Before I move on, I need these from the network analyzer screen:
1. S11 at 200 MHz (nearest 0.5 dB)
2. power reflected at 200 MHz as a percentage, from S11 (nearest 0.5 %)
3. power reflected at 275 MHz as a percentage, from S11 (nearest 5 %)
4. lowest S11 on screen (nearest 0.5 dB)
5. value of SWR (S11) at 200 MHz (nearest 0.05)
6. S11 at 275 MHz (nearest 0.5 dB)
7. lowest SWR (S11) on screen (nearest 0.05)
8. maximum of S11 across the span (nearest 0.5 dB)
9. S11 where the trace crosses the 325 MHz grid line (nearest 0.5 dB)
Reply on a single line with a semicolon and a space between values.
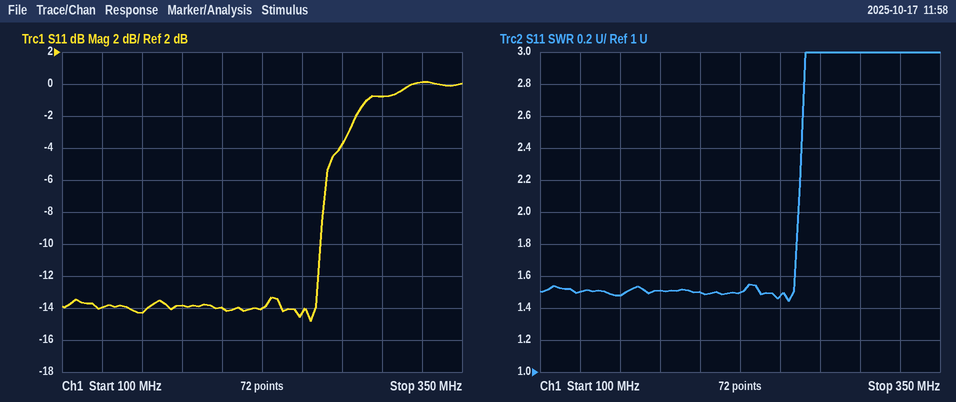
-14.0 dB; 4.0 %; 40 %; -15.0 dB; 1.50; -4.0 dB; 1.45; 0.0 dB; 0.0 dB
